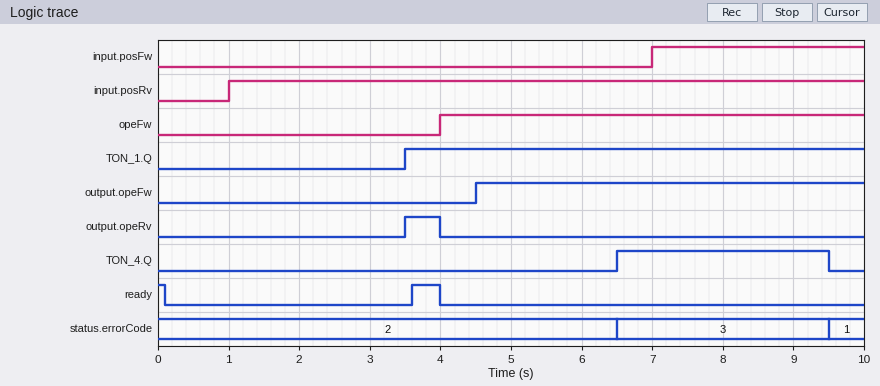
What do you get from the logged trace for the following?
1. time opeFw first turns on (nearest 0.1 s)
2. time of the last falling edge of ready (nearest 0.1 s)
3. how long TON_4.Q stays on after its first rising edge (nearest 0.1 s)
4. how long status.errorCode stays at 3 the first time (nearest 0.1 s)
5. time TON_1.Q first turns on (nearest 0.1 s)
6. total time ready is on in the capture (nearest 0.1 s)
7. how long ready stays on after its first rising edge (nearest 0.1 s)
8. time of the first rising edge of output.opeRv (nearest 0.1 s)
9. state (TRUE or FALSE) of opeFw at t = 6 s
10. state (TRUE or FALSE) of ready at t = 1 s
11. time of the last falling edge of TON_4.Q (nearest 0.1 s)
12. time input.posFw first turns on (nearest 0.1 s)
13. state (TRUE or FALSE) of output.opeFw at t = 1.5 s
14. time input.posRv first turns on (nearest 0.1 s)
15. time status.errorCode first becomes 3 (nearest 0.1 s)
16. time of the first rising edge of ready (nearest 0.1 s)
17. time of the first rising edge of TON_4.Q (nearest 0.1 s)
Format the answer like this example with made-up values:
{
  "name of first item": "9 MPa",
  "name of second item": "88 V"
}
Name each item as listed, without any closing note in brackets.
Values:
{
  "time opeFw first turns on": "4.0 s",
  "time of the last falling edge of ready": "4.0 s",
  "how long TON_4.Q stays on after its first rising edge": "3.0 s",
  "how long status.errorCode stays at 3 the first time": "3.0 s",
  "time TON_1.Q first turns on": "3.5 s",
  "total time ready is on in the capture": "0.5 s",
  "how long ready stays on after its first rising edge": "0.4 s",
  "time of the first rising edge of output.opeRv": "3.5 s",
  "state (TRUE or FALSE) of opeFw at t = 6 s": "TRUE",
  "state (TRUE or FALSE) of ready at t = 1 s": "FALSE",
  "time of the last falling edge of TON_4.Q": "9.5 s",
  "time input.posFw first turns on": "7.0 s",
  "state (TRUE or FALSE) of output.opeFw at t = 1.5 s": "FALSE",
  "time input.posRv first turns on": "1.0 s",
  "time status.errorCode first becomes 3": "6.5 s",
  "time of the first rising edge of ready": "3.6 s",
  "time of the first rising edge of TON_4.Q": "6.5 s"
}
